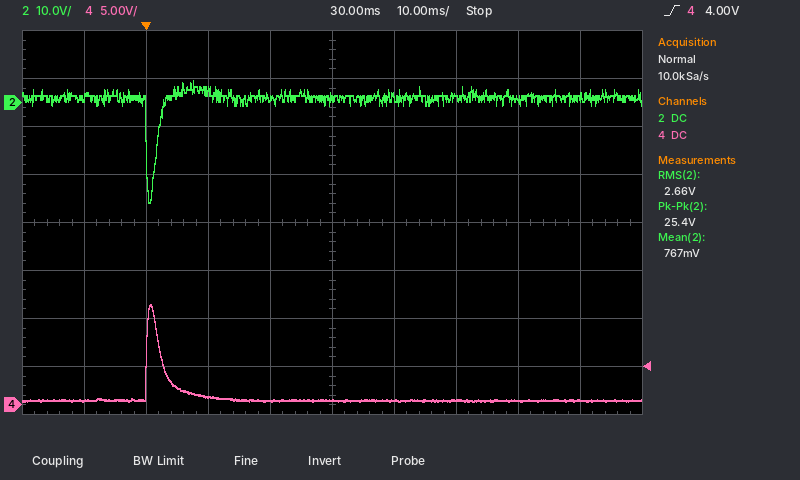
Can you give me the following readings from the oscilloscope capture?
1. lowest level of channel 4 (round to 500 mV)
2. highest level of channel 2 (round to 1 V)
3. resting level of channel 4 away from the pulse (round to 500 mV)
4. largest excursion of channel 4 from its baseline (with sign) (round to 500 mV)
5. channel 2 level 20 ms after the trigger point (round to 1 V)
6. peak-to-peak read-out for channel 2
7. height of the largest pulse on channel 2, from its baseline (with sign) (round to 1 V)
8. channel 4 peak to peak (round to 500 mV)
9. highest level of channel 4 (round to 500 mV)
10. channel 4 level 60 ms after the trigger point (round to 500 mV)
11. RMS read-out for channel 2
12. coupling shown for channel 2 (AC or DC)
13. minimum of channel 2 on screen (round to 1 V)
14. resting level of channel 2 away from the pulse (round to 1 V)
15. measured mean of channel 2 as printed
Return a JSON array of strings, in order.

["500 mV", "5 V", "500 mV", "+10.0 V", "1 V", "25.4 V", "-22 V", "10.0 V", "10.5 V", "500 mV", "2.66 V", "DC", "-21 V", "1 V", "767 mV"]
